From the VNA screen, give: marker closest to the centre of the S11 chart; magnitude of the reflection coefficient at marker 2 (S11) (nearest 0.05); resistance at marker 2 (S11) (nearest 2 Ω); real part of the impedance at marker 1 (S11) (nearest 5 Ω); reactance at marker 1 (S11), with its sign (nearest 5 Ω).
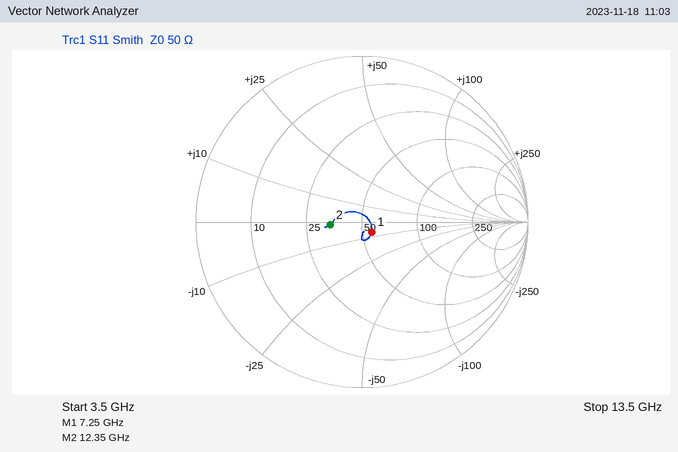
marker 1
0.20
34 Ω
55 Ω
-5 Ω
